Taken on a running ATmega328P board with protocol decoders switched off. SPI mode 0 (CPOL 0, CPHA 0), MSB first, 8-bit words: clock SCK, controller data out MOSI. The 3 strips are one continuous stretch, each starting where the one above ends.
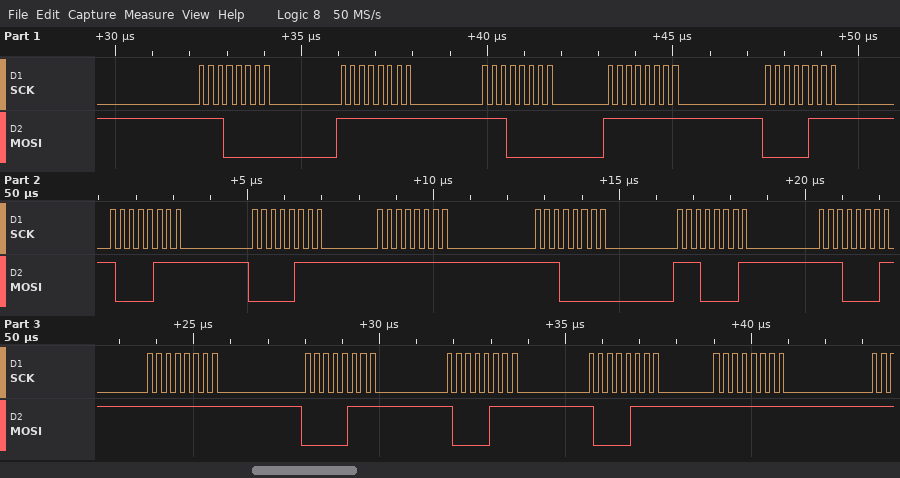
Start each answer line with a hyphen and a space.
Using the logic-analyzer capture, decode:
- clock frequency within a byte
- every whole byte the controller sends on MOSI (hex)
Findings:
- 4 MHz
- 0xE0 0xFF 0xE0 0xFF 0x07 0x87 0x07 0xFF 0xE0 0xE1 0xE1 0xFF 0x07 0x87 0x87 0xFF
